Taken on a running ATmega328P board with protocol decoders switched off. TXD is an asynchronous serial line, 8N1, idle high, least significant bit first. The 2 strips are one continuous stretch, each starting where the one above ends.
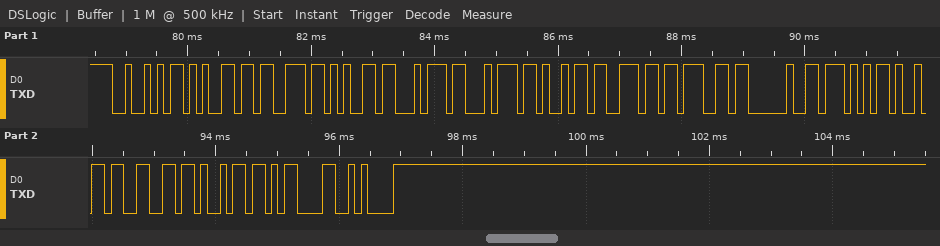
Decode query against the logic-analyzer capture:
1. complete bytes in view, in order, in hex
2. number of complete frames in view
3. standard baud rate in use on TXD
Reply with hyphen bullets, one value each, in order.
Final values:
- 52 65 73 65 74 74 69 6E 67 20 57 69 66 69 0D 0A
- 16
- 9600 baud
